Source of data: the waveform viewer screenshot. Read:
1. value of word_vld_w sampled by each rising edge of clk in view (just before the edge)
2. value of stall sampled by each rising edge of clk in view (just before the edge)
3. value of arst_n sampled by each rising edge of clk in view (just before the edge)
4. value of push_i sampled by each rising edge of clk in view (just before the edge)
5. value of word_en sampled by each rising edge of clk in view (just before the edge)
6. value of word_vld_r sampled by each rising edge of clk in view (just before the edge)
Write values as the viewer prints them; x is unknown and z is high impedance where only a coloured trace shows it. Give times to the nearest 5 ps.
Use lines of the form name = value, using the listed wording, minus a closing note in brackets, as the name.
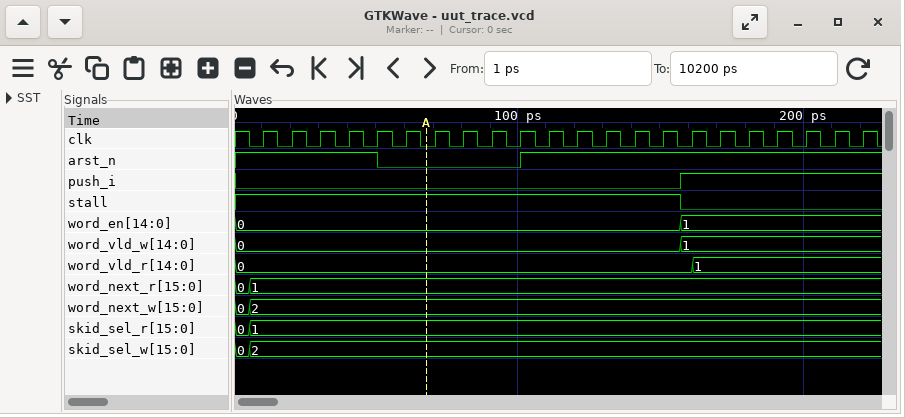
value of word_vld_w sampled by each rising edge of clk in view = 0, 0, 0, 0, 0, 0, 0, 0, 0, 0, 0, 0, 0, 0, 0, 1, 1, 1, 1, 1, 1, 1
value of stall sampled by each rising edge of clk in view = 1 1 1 1 1 1 1 1 1 1 1 1 1 1 1 0 0 0 0 0 0 0
value of arst_n sampled by each rising edge of clk in view = 1 1 1 1 1 0 0 0 0 0 1 1 1 1 1 1 1 1 1 1 1 1
value of push_i sampled by each rising edge of clk in view = 0 0 0 0 0 0 0 0 0 0 0 0 0 0 0 1 1 1 1 1 1 1
value of word_en sampled by each rising edge of clk in view = 0, 0, 0, 0, 0, 0, 0, 0, 0, 0, 0, 0, 0, 0, 0, 1, 1, 1, 1, 1, 1, 1
value of word_vld_r sampled by each rising edge of clk in view = 0, 0, 0, 0, 0, 0, 0, 0, 0, 0, 0, 0, 0, 0, 0, 0, 1, 1, 1, 1, 1, 1
